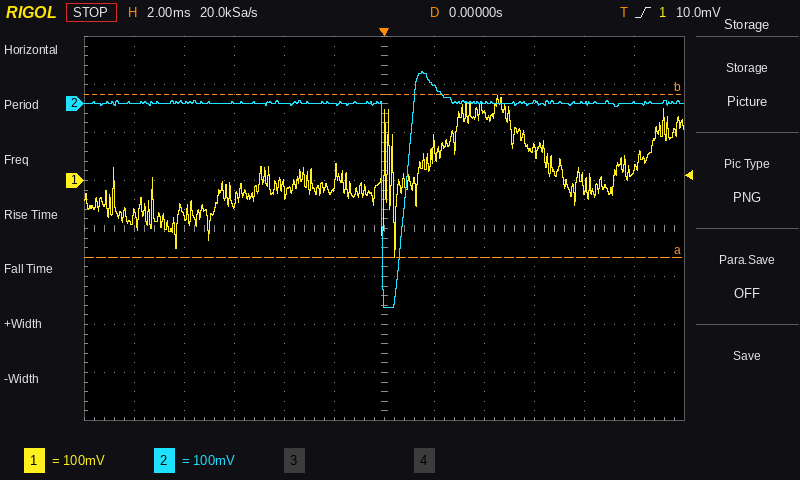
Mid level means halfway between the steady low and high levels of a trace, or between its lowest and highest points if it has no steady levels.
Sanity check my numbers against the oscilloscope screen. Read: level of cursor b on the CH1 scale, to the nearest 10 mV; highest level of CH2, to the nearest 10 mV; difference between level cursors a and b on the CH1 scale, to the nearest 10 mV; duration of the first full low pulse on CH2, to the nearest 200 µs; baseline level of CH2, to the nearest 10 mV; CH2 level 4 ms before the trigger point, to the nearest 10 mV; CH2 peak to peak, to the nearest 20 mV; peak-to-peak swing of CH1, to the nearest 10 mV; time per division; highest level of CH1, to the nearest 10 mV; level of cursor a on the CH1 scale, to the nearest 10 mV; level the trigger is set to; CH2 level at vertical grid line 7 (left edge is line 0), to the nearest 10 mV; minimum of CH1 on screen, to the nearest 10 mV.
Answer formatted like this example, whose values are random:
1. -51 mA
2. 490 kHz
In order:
1. 180 mV
2. 70 mV
3. 340 mV
4. 1.0 ms
5. 0 mV
6. 0 mV
7. 500 mV
8. 340 mV
9. 2 ms
10. 180 mV
11. -160 mV
12. 10.0 mV
13. 40 mV
14. -160 mV
